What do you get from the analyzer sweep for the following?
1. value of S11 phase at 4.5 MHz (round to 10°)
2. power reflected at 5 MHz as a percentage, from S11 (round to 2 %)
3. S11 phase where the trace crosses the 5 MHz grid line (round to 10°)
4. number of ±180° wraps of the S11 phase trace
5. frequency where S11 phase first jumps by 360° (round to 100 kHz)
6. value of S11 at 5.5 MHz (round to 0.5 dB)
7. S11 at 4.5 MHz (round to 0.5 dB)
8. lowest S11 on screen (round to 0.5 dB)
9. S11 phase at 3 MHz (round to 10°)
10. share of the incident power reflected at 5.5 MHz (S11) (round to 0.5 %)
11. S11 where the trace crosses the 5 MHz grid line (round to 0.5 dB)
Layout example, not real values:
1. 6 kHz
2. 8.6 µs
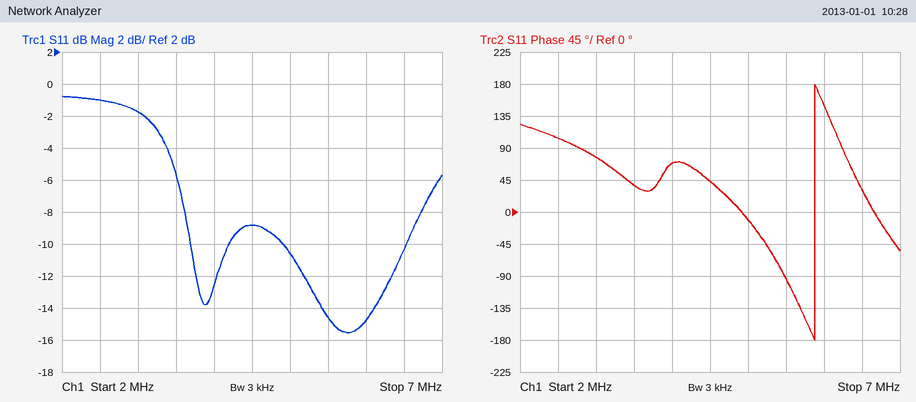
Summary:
1. 40°
2. 8 %
3. -10°
4. 1
5. 5.9 MHz
6. -14.5 dB
7. -9.0 dB
8. -15.5 dB
9. 80°
10. 3.5 %
11. -10.5 dB
